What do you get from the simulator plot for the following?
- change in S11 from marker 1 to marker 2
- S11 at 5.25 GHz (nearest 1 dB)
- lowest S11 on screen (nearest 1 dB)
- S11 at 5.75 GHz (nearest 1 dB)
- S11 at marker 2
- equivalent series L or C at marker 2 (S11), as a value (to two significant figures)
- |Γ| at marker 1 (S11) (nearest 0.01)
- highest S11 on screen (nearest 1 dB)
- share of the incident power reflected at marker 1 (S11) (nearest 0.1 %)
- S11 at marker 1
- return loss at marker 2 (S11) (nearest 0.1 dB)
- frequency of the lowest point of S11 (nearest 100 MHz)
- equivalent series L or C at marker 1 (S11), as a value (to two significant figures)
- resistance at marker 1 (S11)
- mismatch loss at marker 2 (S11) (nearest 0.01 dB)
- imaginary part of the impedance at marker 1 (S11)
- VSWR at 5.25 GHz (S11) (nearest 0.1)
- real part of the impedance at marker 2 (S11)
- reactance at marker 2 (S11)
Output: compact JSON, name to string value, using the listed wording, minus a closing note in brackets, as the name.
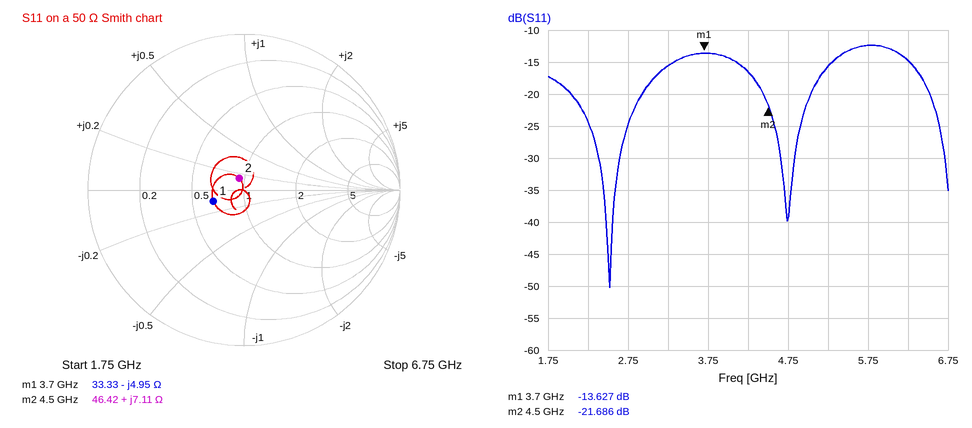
{"change in S11 from marker 1 to marker 2": "-8.059 dB", "S11 at 5.25 GHz": "-16 dB", "lowest S11 on screen": "-50 dB", "S11 at 5.75 GHz": "-12 dB", "S11 at marker 2": "-21.686 dB", "equivalent series L or C at marker 2 (S11), as a value": "250 pH", "|Γ| at marker 1 (S11)": "0.21", "highest S11 on screen": "-12 dB", "share of the incident power reflected at marker 1 (S11)": "4.3 %", "S11 at marker 1": "-13.627 dB", "return loss at marker 2 (S11)": "21.7 dB", "frequency of the lowest point of S11": "2.5 GHz", "equivalent series L or C at marker 1 (S11), as a value": "8.7 pF", "resistance at marker 1": "33.33 Ω", "mismatch loss at marker 2 (S11)": "0.03 dB", "imaginary part of the impedance at marker 1": "-4.95 Ω", "VSWR at 5.25 GHz (S11)": "1.4", "real part of the impedance at marker 2": "46.42 Ω", "reactance at marker 2": "+7.11 Ω"}
